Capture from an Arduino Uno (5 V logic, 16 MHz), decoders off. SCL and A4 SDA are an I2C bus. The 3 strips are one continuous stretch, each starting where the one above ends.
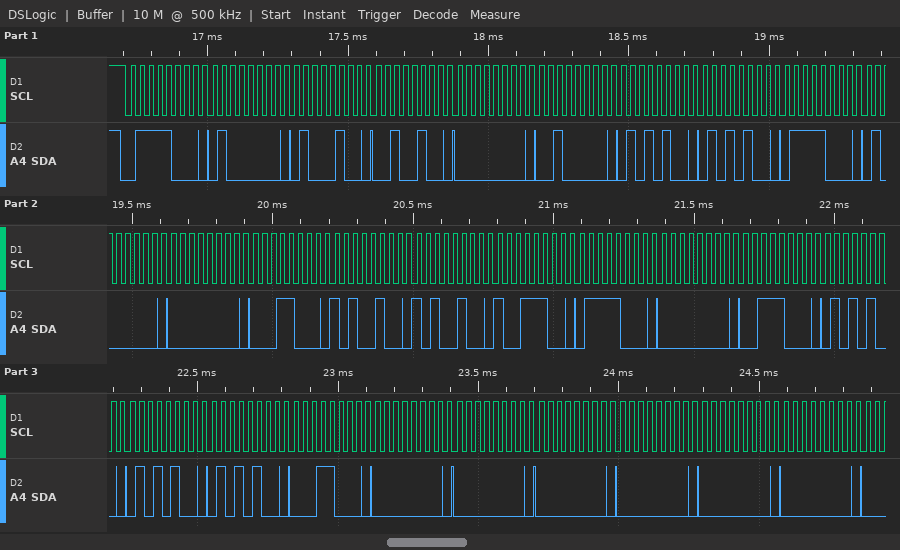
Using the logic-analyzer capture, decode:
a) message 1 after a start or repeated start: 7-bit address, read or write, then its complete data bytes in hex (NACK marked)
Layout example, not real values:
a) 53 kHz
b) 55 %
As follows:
a) 0x3C write: 40 44 24 00 20 54 54 78 40 00 18 A4 A4 9C 78 00 38 54 54 54 18 00 00 00 00 00 00
